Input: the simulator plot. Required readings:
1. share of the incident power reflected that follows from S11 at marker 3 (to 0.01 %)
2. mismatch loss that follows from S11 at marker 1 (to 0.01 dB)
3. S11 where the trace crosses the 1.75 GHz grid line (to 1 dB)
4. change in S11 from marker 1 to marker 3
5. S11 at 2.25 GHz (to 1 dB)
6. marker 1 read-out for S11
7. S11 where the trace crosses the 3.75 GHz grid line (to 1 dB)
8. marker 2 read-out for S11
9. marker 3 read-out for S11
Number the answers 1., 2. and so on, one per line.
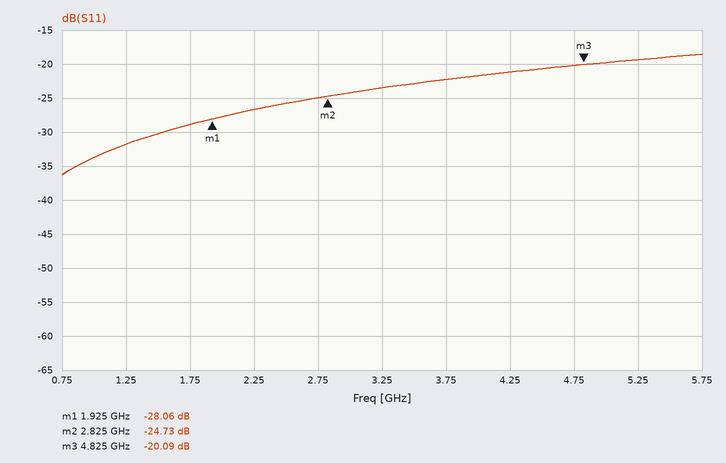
1. 0.98 %
2. 0.01 dB
3. -29 dB
4. 7.97 dB
5. -27 dB
6. -28.06 dB
7. -22 dB
8. -24.73 dB
9. -20.09 dB
